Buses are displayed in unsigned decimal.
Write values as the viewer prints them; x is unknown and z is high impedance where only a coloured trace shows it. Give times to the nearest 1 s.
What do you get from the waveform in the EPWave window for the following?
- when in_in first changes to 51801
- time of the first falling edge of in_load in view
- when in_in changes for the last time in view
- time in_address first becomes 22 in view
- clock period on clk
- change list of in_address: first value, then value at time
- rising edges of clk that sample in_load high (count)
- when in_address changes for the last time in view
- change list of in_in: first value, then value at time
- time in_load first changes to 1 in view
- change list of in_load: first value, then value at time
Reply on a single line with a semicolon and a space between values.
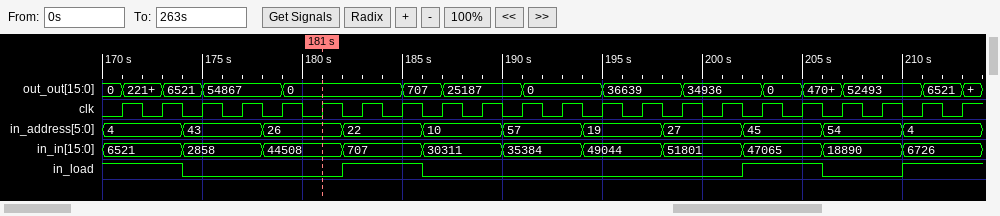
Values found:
198 s; 174 s; 210 s; 182 s; 2 s; 4, 43 at 174 s, 26 at 178 s, 22 at 182 s, 10 at 186 s, 57 at 190 s, 19 at 194 s, 27 at 198 s, 45 at 202 s, 54 at 206 s, 4 at 210 s; 8; 210 s; 6521, 2858 at 174 s, 44508 at 178 s, 707 at 182 s, 30311 at 186 s, 35384 at 190 s, 49044 at 194 s, 51801 at 198 s, 47065 at 202 s, 18890 at 206 s, 6726 at 210 s; 182 s; 1, 0 at 174 s, 1 at 182 s, 0 at 186 s, 1 at 202 s, 0 at 206 s, 1 at 210 s
